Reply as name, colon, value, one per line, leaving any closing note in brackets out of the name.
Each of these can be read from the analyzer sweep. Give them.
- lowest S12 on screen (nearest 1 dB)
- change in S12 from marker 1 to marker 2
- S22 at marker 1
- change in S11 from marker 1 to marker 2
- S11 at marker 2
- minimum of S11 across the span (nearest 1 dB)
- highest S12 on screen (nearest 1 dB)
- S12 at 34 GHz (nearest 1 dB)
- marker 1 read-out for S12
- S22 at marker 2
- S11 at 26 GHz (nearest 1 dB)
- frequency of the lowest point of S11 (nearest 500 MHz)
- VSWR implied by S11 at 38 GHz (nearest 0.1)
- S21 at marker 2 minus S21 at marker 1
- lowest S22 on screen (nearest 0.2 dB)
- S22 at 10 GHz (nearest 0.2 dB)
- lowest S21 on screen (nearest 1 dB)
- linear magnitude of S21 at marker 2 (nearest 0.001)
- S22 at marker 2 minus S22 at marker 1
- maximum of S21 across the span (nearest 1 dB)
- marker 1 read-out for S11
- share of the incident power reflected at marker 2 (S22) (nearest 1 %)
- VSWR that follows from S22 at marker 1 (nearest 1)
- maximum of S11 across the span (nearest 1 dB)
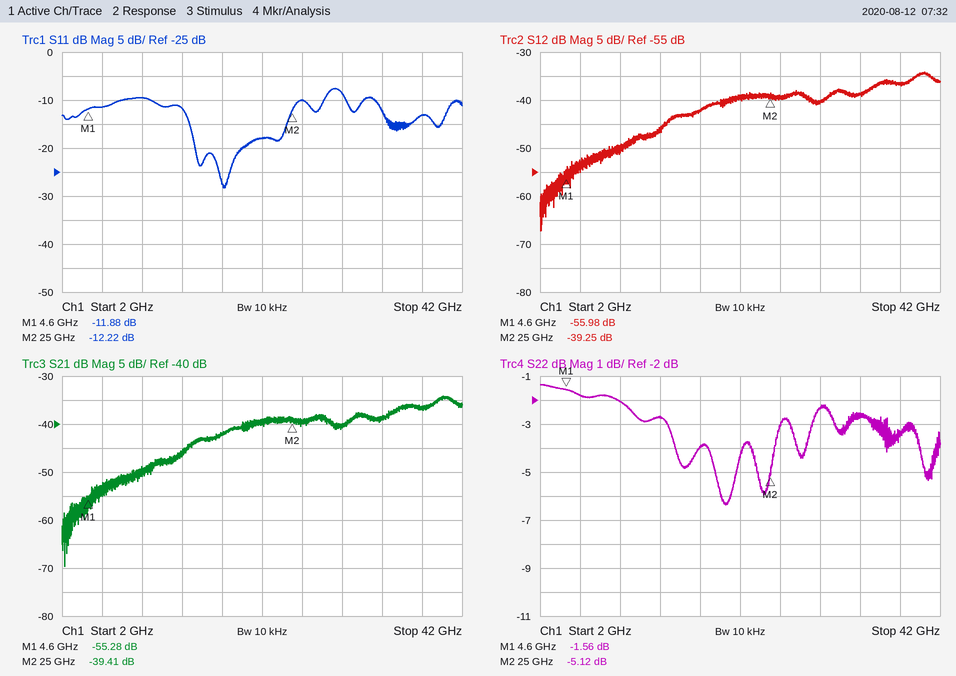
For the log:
lowest S12 on screen: -67 dB
change in S12 from marker 1 to marker 2: 16.73 dB
S22 at marker 1: -1.56 dB
change in S11 from marker 1 to marker 2: -0.34 dB
S11 at marker 2: -12.22 dB
minimum of S11 across the span: -28 dB
highest S12 on screen: -34 dB
S12 at 34 GHz: -39 dB
marker 1 read-out for S12: -55.98 dB
S22 at marker 2: -5.12 dB
S11 at 26 GHz: -10 dB
frequency of the lowest point of S11: 18.0 GHz
VSWR implied by S11 at 38 GHz: 1.6
S21 at marker 2 minus S21 at marker 1: 15.87 dB
lowest S22 on screen: -6.4 dB
S22 at 10 GHz: -2.0 dB
lowest S21 on screen: -70 dB
linear magnitude of S21 at marker 2: 0.011
S22 at marker 2 minus S22 at marker 1: -3.56 dB
maximum of S21 across the span: -34 dB
marker 1 read-out for S11: -11.88 dB
share of the incident power reflected at marker 2 (S22): 31 %
VSWR that follows from S22 at marker 1: 11
maximum of S11 across the span: -8 dB
